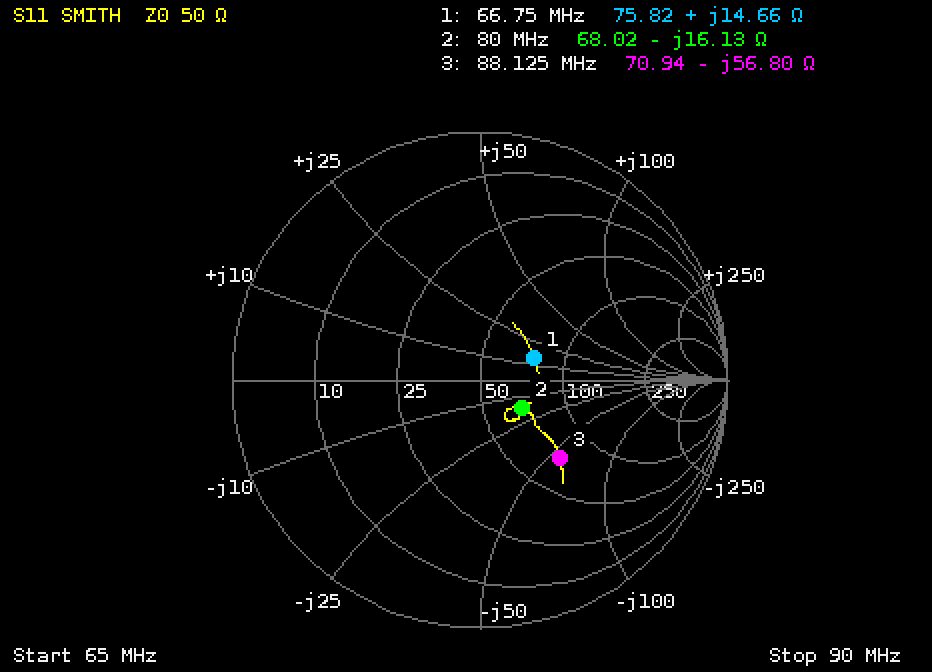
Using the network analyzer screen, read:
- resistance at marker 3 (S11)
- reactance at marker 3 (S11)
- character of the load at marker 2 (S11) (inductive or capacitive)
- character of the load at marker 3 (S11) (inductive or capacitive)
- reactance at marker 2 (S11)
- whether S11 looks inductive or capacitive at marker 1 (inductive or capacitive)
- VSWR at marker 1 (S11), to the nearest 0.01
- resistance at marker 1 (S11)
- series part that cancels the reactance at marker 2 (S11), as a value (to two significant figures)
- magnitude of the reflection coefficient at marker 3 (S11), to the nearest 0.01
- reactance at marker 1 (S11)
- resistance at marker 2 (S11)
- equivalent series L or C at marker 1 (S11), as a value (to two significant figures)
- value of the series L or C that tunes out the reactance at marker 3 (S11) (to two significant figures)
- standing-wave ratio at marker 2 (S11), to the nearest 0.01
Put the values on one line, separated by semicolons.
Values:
70.94 Ω; -56.80 Ω; capacitive; capacitive; -16.13 Ω; inductive; 1.61; 75.82 Ω; 32 nH; 0.45; +14.66 Ω; 68.02 Ω; 35 nH; 100 nH; 1.51
